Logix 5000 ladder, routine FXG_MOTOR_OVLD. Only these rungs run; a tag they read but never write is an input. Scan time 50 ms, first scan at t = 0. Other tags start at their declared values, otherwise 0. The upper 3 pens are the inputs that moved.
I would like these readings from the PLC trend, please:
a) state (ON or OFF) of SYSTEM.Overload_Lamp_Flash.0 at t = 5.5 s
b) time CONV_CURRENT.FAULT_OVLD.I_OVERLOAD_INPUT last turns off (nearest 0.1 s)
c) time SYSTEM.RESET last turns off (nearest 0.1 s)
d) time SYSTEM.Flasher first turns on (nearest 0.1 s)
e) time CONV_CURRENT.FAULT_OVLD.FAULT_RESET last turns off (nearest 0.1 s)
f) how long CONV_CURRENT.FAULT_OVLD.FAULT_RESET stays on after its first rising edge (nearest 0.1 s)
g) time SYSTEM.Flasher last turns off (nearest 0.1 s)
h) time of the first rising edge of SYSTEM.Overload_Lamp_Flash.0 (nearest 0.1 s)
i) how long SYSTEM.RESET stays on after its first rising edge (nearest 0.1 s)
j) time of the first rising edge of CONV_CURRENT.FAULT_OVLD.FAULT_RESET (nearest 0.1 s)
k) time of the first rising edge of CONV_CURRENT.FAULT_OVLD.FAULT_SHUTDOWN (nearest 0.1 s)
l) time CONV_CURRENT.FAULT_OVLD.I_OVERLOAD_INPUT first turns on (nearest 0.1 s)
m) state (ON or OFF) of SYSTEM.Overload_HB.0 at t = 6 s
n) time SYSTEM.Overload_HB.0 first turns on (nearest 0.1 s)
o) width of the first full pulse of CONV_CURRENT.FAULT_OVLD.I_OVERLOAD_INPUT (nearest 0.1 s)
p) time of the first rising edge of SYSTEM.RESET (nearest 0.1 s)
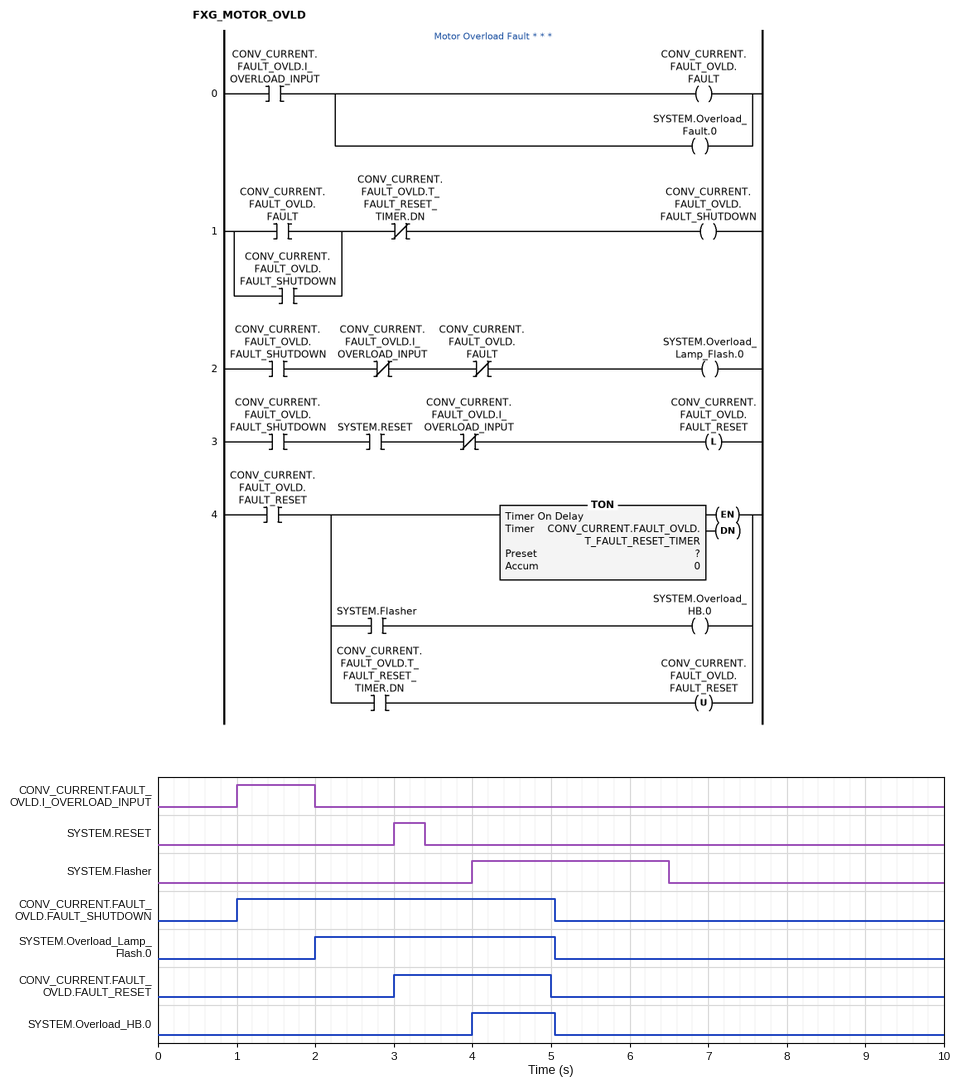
OFF
2.0 s
3.4 s
4.0 s
5.0 s
2.0 s
6.5 s
2.0 s
0.4 s
3.0 s
1.0 s
1.0 s
OFF
4.0 s
1.0 s
3.0 s
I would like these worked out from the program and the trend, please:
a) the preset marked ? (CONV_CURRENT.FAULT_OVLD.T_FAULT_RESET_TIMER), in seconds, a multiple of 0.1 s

2.0 s
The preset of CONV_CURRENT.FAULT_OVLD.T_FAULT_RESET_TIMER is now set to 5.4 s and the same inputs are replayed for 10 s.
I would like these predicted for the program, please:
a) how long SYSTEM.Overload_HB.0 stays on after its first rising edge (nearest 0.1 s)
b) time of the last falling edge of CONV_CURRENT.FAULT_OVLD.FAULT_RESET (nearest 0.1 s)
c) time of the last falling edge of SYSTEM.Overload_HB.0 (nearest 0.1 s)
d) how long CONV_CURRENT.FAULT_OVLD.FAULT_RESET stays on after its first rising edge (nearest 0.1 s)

2.5 s
8.4 s
6.5 s
5.4 s
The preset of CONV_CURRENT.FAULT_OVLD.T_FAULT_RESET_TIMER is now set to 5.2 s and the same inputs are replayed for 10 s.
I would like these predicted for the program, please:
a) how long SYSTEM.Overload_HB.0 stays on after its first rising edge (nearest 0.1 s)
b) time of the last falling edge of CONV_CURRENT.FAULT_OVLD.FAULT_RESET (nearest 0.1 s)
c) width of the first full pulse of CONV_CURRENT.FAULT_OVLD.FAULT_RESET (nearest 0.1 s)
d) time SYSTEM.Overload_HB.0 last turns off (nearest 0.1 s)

2.5 s
8.2 s
5.2 s
6.5 s
